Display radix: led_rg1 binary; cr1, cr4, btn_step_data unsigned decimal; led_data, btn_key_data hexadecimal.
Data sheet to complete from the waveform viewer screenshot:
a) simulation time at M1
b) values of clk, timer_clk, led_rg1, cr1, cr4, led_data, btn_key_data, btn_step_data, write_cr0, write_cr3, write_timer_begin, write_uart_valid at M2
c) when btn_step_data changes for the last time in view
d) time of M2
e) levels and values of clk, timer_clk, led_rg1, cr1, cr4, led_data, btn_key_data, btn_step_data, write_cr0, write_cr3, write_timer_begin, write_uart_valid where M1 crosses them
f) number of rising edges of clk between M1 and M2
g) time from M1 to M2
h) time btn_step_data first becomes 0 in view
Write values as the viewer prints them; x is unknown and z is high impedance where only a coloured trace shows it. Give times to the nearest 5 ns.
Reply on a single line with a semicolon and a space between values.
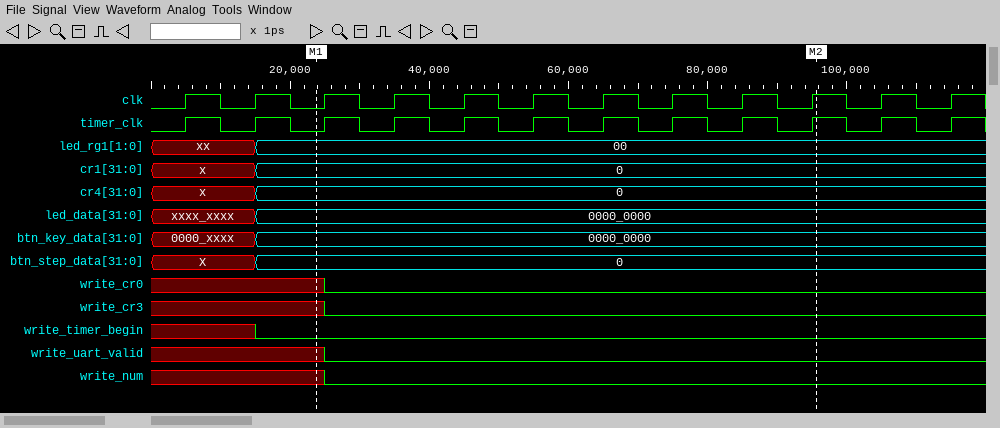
25 ns; clk=1, timer_clk=1, led_rg1=00, cr1=0, cr4=0, led_data=0000_0000, btn_key_data=0000_0000, btn_step_data=0, write_cr0=0, write_cr3=0, write_timer_begin=0, write_uart_valid=0; 15 ns; 95 ns; clk=0, timer_clk=0, led_rg1=00, cr1=0, cr4=0, led_data=0000_0000, btn_key_data=0000_0000, btn_step_data=0, write_cr0=x, write_cr3=x, write_timer_begin=0, write_uart_valid=x; 8; 70 ns; 15 ns
